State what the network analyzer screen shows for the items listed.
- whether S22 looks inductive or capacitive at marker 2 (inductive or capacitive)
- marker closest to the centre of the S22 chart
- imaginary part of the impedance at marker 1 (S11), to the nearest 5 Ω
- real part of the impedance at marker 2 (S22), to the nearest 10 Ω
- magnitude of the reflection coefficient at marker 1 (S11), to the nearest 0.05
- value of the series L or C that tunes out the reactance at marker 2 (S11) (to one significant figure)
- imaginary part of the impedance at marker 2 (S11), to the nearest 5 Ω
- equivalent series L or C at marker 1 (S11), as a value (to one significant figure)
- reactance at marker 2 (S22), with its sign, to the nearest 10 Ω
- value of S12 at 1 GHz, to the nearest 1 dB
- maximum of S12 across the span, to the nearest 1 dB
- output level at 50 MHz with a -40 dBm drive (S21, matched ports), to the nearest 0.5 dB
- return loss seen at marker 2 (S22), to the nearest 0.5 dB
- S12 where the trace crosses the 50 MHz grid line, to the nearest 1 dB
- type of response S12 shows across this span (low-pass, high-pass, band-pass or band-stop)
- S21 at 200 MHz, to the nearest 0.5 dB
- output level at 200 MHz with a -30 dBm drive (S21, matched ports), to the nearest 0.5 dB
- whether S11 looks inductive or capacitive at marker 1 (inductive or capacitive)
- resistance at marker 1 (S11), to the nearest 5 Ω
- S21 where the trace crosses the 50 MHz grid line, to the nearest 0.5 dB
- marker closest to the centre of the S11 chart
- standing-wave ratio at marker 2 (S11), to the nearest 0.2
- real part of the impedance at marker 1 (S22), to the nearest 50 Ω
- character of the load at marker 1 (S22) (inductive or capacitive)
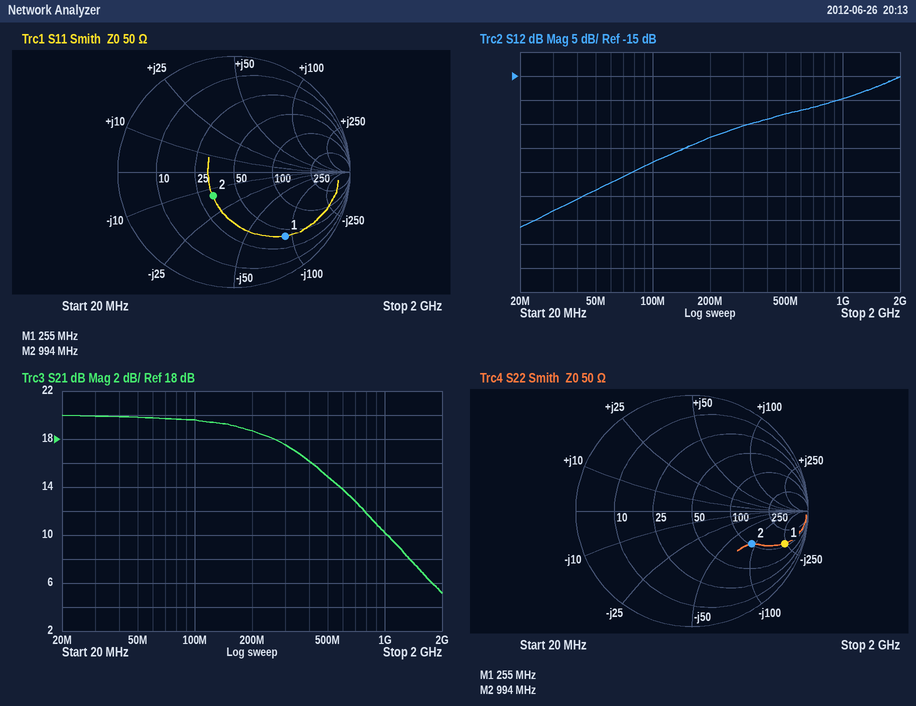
capacitive
marker 2
-90 Ω
100 Ω
0.70
2 nH
-15 Ω
7 pF
-90 Ω
-20 dB
-15 dB
-20.0 dBm
4.5 dB
-39 dB
high-pass
18.5 dB
-11.5 dBm
capacitive
40 Ω
20.0 dB
marker 2
1.8
100 Ω
capacitive
